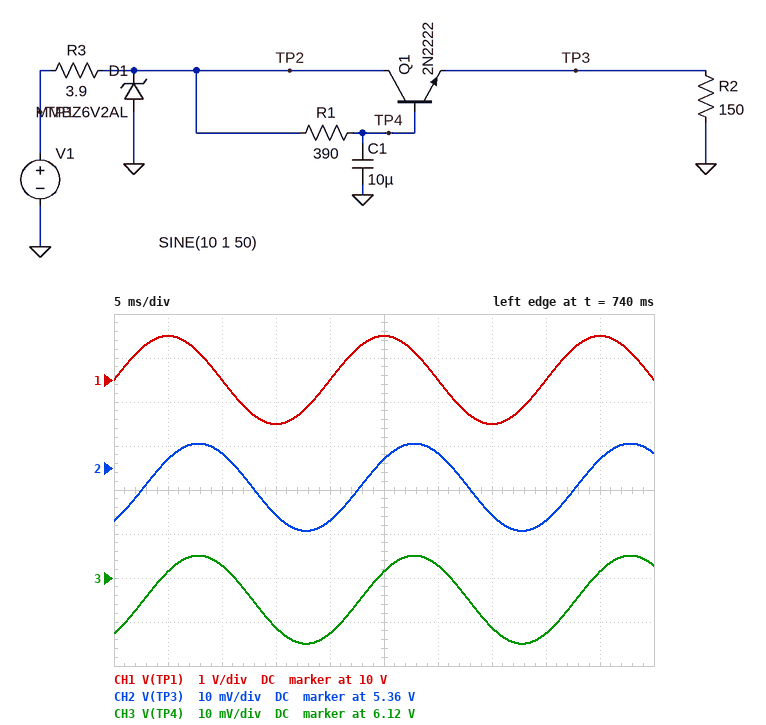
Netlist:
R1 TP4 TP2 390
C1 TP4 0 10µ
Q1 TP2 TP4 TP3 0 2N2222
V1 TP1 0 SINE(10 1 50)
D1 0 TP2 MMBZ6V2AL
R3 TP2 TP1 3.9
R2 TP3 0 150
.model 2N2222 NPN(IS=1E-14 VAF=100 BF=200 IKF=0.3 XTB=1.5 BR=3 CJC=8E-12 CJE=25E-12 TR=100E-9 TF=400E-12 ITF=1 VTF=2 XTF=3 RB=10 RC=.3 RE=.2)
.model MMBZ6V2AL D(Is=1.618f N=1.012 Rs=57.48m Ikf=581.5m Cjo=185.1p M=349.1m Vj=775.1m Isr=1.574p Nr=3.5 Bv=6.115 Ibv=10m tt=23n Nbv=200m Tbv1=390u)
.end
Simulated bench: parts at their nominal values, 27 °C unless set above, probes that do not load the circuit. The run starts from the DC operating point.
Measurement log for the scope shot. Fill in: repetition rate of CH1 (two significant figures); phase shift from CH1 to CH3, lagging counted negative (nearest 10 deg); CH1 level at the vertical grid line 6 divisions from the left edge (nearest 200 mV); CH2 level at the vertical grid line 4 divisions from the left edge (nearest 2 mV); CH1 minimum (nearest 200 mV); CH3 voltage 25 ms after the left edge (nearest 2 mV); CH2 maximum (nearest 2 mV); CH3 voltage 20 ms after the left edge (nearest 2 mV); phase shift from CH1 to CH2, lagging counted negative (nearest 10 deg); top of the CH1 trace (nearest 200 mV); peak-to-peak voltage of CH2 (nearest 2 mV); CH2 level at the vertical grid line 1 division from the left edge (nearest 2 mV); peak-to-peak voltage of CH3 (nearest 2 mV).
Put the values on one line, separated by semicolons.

50 Hz; -50 deg; 10.0 V; 5.348 V; 9.0 V; 6.122 V; 5.366 V; 6.108 V; -50 deg; 11.0 V; 20 mV; 5.362 V; 20 mV
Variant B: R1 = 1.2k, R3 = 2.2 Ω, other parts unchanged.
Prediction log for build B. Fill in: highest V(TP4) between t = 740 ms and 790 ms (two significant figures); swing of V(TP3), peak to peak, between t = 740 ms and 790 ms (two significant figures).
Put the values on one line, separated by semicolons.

6.0 V; 14 mV
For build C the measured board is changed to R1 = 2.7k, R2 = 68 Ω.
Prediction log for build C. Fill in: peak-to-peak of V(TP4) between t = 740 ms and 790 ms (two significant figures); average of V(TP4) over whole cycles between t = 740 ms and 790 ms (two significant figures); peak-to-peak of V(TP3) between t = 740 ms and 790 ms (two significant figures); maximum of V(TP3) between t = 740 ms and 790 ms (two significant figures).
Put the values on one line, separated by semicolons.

3.8 mV; 5.2 V; 3.7 mV; 4.4 V
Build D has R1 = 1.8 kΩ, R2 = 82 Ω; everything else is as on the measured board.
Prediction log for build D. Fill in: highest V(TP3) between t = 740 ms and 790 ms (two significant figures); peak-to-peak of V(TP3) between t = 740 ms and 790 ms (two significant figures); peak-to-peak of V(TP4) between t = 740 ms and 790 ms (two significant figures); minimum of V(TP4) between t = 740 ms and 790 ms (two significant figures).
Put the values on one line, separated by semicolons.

4.8 V; 5.5 mV; 5.6 mV; 5.6 V
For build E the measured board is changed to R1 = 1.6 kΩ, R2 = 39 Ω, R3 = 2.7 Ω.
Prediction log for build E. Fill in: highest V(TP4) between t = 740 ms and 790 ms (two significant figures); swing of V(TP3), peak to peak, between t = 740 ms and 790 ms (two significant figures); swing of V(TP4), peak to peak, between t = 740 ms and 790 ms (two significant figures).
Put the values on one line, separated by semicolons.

5.1 V; 8.6 mV; 8.7 mV
